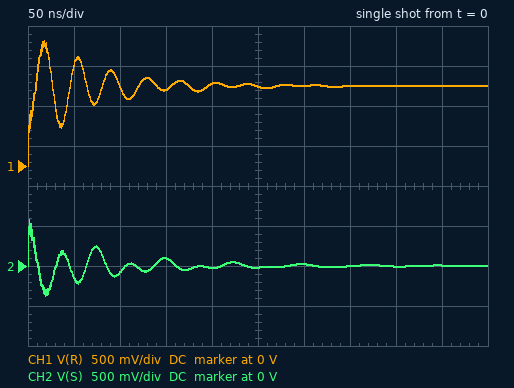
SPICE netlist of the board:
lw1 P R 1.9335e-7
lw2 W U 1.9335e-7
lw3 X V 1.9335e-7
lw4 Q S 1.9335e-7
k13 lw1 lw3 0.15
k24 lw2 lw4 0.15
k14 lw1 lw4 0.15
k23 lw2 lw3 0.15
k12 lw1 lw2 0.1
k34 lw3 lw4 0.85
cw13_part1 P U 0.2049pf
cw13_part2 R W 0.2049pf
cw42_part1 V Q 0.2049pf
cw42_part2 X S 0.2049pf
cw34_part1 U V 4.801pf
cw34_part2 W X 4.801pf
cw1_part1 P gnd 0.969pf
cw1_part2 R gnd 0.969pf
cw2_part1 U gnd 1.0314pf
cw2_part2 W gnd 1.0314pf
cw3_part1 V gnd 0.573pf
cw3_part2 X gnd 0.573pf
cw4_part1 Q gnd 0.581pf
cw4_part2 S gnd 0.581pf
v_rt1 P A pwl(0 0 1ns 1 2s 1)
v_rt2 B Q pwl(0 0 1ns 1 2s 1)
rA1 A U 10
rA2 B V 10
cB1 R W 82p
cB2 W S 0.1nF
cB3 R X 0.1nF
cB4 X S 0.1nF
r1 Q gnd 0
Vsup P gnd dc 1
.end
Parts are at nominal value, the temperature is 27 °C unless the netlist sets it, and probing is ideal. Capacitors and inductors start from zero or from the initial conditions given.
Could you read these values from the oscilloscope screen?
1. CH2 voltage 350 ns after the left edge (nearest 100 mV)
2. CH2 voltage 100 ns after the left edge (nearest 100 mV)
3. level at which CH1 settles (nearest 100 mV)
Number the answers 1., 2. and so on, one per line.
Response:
1. 0 V
2. -100 mV
3. 1.0 V
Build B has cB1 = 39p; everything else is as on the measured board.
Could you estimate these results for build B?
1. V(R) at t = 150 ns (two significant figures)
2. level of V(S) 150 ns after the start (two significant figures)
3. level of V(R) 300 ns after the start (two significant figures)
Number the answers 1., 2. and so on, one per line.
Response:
1. 650 mV
2. 210 mV
3. 790 mV
